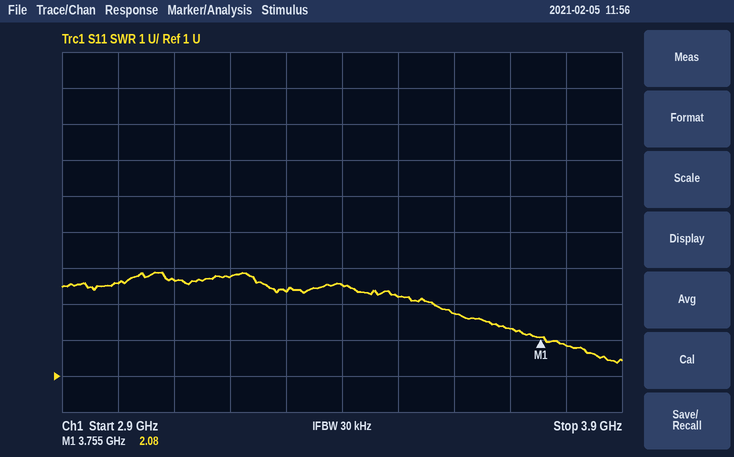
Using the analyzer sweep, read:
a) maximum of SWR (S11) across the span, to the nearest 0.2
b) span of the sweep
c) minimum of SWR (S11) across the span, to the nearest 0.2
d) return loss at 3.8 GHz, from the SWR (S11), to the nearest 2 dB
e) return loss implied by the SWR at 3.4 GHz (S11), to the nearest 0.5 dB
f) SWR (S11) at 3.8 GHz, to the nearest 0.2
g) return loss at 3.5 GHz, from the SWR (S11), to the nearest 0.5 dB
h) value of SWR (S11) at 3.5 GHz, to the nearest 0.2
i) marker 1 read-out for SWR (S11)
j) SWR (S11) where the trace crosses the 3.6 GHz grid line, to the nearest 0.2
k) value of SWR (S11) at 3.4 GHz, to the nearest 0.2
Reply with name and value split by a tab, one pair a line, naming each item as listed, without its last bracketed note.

maximum of SWR (S11) across the span, to the nearest 0.2	3.8
span of the sweep	1 GHz
minimum of SWR (S11) across the span, to the nearest 0.2	1.4
return loss at 3.8 GHz, from the SWR (S11), to the nearest 2 dB	10 dB
return loss implied by the SWR at 3.4 GHz (S11), to the nearest 0.5 dB	5.0 dB
SWR (S11) at 3.8 GHz, to the nearest 0.2	1.8
return loss at 3.5 GHz, from the SWR (S11), to the nearest 0.5 dB	5.5 dB
value of SWR (S11) at 3.5 GHz, to the nearest 0.2	3.2
marker 1 read-out for SWR	2.08
SWR (S11) where the trace crosses the 3.6 GHz grid line, to the nearest 0.2	2.8
value of SWR (S11) at 3.4 GHz, to the nearest 0.2	3.6
